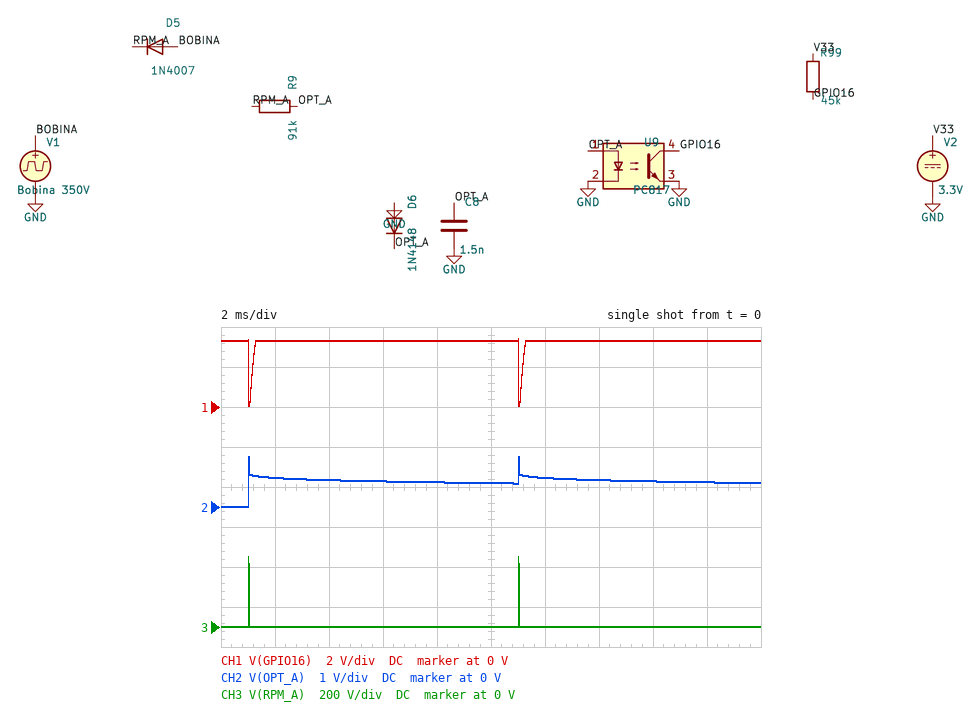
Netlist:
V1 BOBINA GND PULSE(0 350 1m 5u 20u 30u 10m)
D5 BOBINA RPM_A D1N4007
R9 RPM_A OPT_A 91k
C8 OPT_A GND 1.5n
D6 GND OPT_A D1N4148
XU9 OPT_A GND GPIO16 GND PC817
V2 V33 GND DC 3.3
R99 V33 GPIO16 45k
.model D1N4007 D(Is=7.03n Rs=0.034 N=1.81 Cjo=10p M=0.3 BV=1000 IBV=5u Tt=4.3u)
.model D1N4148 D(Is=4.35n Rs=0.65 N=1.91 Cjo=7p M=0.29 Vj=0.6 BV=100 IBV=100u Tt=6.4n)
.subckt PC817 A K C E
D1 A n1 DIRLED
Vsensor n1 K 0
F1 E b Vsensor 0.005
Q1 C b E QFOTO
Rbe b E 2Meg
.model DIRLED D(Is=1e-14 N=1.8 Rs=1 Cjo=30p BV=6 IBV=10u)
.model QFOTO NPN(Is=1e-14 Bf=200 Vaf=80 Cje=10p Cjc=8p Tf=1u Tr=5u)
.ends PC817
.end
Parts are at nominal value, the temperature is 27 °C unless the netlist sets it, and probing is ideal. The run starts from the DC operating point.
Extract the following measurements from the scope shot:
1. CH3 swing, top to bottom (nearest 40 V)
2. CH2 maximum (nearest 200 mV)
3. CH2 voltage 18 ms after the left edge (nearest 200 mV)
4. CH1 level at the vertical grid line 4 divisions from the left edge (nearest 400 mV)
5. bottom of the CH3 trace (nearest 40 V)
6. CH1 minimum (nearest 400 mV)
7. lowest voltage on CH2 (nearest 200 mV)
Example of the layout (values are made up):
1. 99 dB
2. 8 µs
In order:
1. 360 V
2. 1.2 V
3. 600 mV
4. 3.2 V
5. 0 V
6. 0 V
7. 0 V
